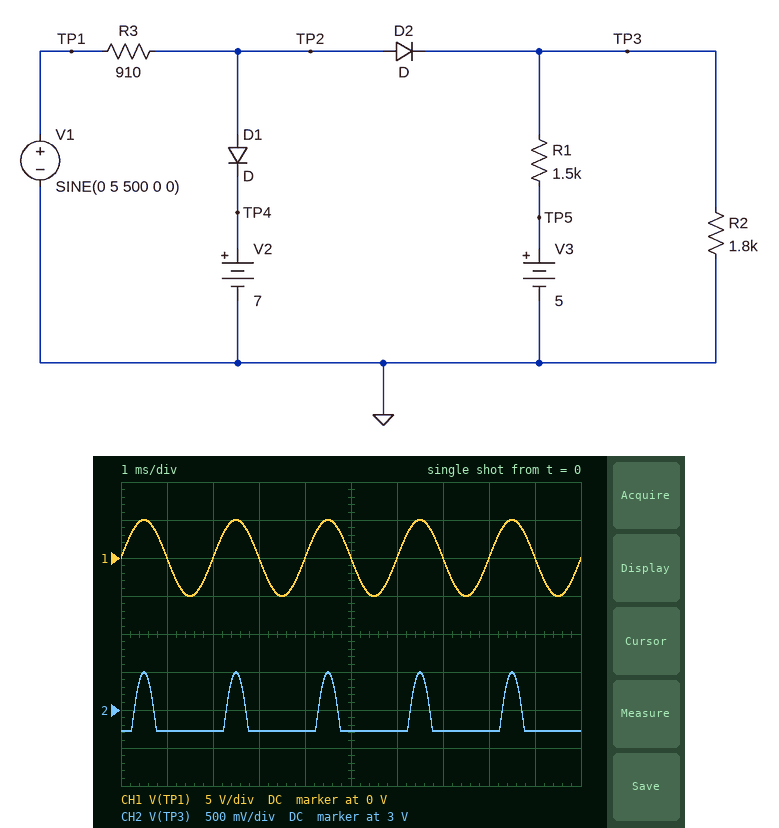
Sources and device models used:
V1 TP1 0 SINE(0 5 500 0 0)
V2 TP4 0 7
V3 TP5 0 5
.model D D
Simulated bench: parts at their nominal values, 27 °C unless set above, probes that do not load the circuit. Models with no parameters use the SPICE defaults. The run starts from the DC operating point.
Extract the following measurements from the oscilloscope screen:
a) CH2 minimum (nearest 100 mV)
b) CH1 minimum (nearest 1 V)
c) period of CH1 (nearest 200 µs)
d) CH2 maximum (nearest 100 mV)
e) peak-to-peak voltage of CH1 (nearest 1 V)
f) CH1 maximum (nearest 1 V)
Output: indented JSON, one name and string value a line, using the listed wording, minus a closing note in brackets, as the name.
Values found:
{
  "CH2 minimum": "2.7 V",
  "CH1 minimum": "-5 V",
  "period of CH1": "2.0 ms",
  "CH2 maximum": "3.5 V",
  "peak-to-peak voltage of CH1": "10 V",
  "CH1 maximum": "5 V"
}
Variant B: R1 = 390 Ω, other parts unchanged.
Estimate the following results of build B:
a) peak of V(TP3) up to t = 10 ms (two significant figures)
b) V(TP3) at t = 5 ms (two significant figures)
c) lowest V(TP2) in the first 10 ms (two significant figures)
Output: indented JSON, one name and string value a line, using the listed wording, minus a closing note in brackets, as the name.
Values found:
{
  "peak of V(TP3) up to t = 10 ms": "4.2 V",
  "V(TP3) at t = 5 ms": "4.1 V",
  "lowest V(TP2) in the first 10 ms": "-5.0 V"
}
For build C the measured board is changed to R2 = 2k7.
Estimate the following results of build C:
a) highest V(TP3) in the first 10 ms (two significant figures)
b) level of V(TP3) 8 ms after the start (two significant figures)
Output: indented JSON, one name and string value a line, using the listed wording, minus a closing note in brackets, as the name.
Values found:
{
  "highest V(TP3) in the first 10 ms": "3.8 V",
  "level of V(TP3) 8 ms after the start": "3.2 V"
}
